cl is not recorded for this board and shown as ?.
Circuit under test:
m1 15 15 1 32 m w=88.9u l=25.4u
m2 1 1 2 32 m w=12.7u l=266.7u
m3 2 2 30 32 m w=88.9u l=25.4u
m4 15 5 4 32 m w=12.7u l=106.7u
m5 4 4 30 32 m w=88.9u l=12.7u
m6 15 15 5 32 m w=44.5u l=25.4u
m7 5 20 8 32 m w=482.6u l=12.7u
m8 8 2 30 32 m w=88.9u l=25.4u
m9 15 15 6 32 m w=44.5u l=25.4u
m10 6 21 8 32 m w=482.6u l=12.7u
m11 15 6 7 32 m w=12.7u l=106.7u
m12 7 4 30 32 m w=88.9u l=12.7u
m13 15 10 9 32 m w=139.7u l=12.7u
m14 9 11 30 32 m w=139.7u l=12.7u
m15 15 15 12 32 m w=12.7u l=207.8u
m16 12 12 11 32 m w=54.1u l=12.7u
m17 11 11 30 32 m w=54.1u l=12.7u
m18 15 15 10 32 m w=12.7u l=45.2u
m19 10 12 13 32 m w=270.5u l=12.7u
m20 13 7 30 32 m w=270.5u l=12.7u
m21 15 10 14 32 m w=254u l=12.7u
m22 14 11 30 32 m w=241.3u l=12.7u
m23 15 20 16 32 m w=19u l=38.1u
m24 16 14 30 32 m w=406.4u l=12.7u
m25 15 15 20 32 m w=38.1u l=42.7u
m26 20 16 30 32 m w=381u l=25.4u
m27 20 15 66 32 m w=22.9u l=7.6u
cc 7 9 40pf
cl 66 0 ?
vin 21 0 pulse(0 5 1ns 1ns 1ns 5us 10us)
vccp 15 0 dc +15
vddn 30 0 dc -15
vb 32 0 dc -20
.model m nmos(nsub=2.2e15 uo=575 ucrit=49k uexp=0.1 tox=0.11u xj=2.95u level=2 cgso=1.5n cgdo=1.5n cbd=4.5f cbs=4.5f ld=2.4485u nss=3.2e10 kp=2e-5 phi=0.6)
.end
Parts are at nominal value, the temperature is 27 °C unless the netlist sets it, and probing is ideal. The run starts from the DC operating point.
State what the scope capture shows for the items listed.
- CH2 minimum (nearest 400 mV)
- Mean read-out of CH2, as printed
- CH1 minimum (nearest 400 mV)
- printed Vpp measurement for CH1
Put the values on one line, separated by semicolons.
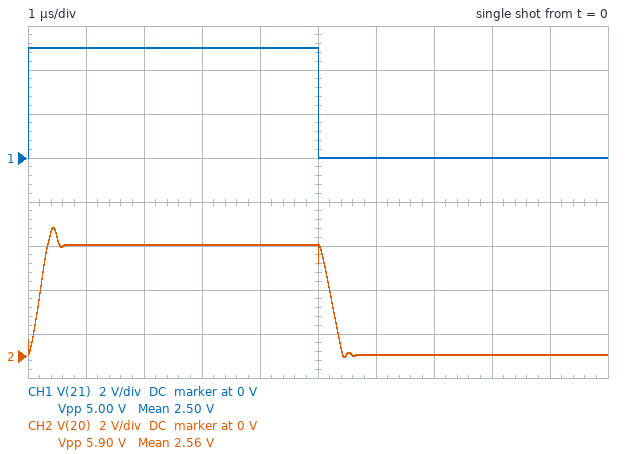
0 V; 2.56 V; 0 V; 5.00 V
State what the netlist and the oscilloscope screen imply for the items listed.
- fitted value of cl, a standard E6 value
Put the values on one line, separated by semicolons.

22 pF
